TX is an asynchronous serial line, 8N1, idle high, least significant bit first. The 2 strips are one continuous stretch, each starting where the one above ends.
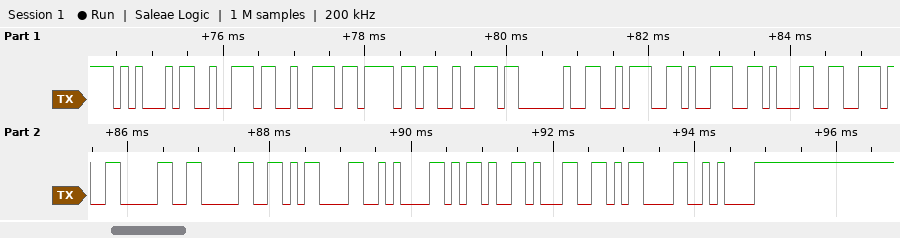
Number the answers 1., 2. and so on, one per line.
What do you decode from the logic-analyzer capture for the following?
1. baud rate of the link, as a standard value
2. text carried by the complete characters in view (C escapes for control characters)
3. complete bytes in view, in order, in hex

1. 9600 baud
2. "Error :91.00\r\n-1\r\n"
3. 0x45 0x72 0x72 0x6F 0x72 0x20 0x3A 0x39 0x31 0x2E 0x30 0x30 0x0D 0x0A 0x2D 0x31 0x0D 0x0A
